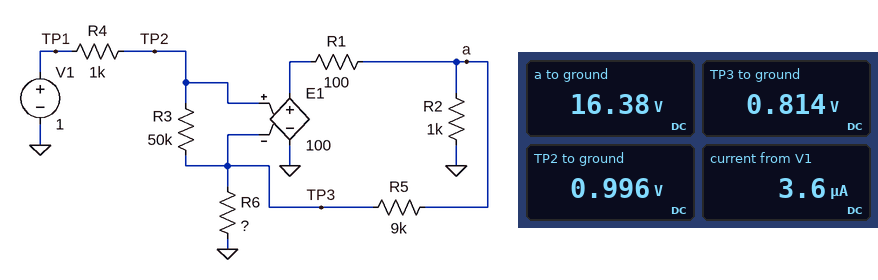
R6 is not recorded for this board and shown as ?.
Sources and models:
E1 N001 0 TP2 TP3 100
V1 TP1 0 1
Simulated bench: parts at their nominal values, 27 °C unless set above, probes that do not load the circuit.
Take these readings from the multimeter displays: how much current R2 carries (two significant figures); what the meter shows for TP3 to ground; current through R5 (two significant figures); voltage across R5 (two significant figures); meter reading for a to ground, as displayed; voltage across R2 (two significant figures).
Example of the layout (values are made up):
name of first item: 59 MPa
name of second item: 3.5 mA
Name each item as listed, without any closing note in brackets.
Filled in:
how much current R2 carries: 16 mA
what the meter shows for TP3 to ground: 0.814 V
current through R5: 1.7 mA
voltage across R5: 16 V
meter reading for a to ground, as displayed: 16.38 V
voltage across R2: 16 V
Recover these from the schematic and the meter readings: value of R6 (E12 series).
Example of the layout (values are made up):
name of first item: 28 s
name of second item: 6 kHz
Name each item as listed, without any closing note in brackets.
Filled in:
value of R6: 470 Ω
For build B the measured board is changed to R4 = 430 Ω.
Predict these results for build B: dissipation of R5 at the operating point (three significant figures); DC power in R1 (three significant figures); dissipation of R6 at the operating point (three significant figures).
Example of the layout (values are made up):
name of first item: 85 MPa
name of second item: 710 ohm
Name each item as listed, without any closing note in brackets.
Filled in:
dissipation of R5 at the operating point: 27.0 mW
DC power in R1: 32.9 mW
dissipation of R6 at the operating point: 1.42 mW
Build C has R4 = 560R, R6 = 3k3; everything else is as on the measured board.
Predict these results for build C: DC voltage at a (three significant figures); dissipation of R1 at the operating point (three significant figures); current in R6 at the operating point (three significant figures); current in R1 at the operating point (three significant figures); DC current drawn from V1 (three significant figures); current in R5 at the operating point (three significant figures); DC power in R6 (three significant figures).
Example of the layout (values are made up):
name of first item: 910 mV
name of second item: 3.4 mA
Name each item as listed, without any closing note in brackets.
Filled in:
DC voltage at a: 3.57 V
dissipation of R1 at the operating point: 1.49 mW
current in R6 at the operating point: 291 µA
current in R1 at the operating point: 3.86 mA
DC current drawn from V1: 791 nA
current in R5 at the operating point: 290 µA
DC power in R6: 279 µW
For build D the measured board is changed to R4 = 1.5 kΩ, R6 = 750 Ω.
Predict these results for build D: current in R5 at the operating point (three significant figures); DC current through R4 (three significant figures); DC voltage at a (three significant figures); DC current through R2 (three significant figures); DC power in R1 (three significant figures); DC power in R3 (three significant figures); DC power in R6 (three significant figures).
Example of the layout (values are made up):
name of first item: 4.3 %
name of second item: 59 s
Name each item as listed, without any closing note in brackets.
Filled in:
current in R5 at the operating point: 1.16 mA
DC current through R4: 2.51 µA
DC voltage at a: 11.3 V
DC current through R2: 11.3 mA
DC power in R1: 15.5 mW
DC power in R3: 315 nW
DC power in R6: 1.01 mW
